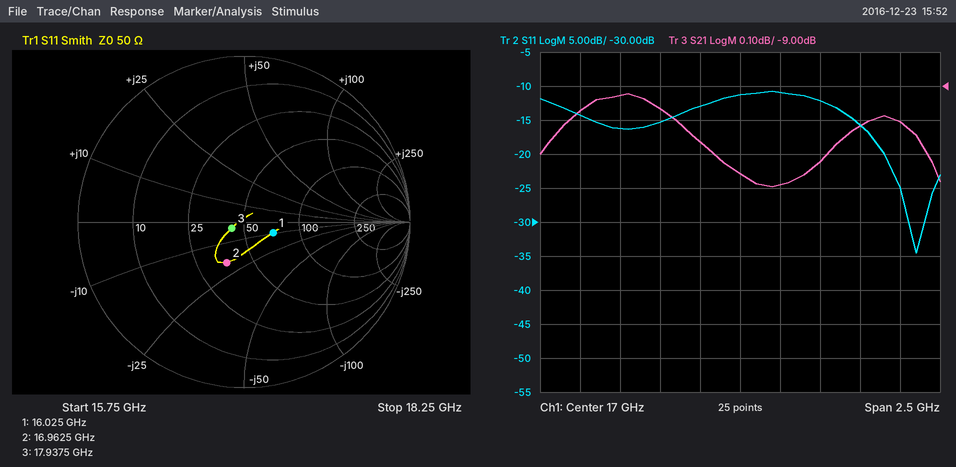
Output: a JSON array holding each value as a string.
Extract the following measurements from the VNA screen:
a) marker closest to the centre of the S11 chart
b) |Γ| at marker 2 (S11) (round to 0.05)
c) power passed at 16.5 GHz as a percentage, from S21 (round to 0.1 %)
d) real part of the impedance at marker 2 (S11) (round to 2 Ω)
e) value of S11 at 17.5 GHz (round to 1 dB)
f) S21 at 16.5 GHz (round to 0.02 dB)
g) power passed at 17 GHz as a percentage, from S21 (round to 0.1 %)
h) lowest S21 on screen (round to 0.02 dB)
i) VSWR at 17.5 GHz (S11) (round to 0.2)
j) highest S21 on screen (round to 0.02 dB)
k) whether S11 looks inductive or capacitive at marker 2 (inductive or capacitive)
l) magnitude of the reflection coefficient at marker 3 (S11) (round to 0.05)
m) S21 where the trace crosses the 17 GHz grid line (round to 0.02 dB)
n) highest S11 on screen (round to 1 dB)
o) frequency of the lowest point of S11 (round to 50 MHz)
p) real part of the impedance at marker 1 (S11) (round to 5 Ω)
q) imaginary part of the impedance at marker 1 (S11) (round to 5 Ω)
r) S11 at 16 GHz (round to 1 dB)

["marker 3", "0.25", "12.4 %", "36 Ω", "-12 dB", "-9.06 dB", "11.9 %", "-9.30 dB", "1.6", "-9.02 dB", "capacitive", "0.10", "-9.26 dB", "-11 dB", "18.10 GHz", "70 Ω", "-10 Ω", "-14 dB"]
